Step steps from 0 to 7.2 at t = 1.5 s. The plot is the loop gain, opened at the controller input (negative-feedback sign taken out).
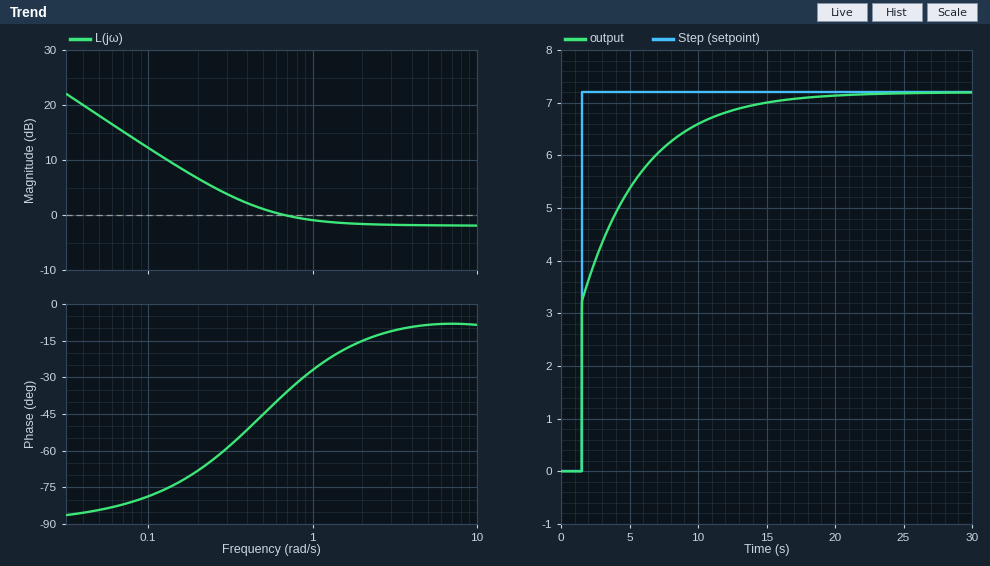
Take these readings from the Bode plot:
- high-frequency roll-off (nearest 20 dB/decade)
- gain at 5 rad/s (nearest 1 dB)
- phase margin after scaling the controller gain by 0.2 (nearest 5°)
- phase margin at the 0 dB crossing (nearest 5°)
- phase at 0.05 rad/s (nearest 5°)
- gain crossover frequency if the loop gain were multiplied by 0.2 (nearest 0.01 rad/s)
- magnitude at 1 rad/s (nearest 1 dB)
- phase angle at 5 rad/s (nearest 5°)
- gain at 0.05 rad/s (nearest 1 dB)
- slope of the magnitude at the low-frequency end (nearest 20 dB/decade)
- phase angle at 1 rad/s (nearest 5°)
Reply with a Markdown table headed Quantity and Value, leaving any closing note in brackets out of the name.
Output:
| Quantity | Value |
|---|---|
| high-frequency roll-off | 0 dB/decade |
| gain at 5 rad/s | -2 dB |
| phase margin after scaling the controller gain by 0.2 | 100° |
| phase margin at the 0 dB crossing | 145° |
| phase at 0.05 rad/s | -85° |
| gain crossover frequency if the loop gain were multiplied by 0.2 | 0.08 rad/s |
| magnitude at 1 rad/s | -1 dB |
| phase angle at 5 rad/s | -10° |
| gain at 0.05 rad/s | 18 dB |
| slope of the magnitude at the low-frequency end | -20 dB/decade |
| phase angle at 1 rad/s | -25° |
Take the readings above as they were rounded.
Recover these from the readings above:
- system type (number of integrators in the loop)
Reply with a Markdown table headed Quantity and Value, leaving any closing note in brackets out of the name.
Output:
| Quantity | Value |
|---|---|
| system type | 1 |
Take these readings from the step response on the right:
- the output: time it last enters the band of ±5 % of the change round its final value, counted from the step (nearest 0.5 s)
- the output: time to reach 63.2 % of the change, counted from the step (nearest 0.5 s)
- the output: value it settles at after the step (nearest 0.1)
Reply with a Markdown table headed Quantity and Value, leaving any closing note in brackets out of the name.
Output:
| Quantity | Value |
|---|---|
| the output: time it last enters the band of ±5 % of the change round its final value, counted from the step | 11.0 s |
| the output: time to reach 63.2 % of the change, counted from the step | 2.0 s |
| the output: value it settles at after the step | 7.2 |
